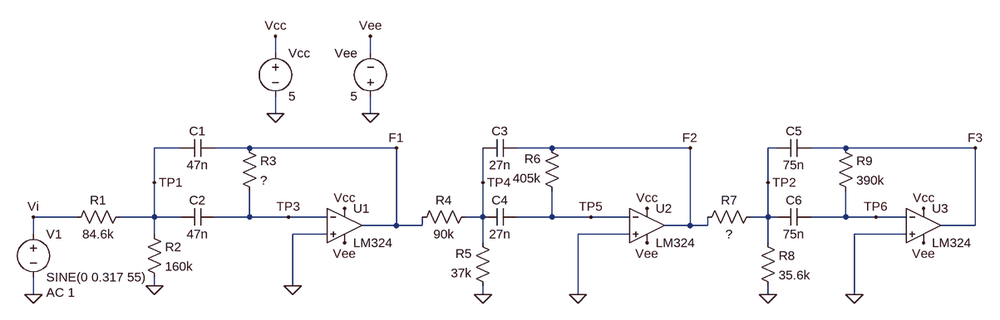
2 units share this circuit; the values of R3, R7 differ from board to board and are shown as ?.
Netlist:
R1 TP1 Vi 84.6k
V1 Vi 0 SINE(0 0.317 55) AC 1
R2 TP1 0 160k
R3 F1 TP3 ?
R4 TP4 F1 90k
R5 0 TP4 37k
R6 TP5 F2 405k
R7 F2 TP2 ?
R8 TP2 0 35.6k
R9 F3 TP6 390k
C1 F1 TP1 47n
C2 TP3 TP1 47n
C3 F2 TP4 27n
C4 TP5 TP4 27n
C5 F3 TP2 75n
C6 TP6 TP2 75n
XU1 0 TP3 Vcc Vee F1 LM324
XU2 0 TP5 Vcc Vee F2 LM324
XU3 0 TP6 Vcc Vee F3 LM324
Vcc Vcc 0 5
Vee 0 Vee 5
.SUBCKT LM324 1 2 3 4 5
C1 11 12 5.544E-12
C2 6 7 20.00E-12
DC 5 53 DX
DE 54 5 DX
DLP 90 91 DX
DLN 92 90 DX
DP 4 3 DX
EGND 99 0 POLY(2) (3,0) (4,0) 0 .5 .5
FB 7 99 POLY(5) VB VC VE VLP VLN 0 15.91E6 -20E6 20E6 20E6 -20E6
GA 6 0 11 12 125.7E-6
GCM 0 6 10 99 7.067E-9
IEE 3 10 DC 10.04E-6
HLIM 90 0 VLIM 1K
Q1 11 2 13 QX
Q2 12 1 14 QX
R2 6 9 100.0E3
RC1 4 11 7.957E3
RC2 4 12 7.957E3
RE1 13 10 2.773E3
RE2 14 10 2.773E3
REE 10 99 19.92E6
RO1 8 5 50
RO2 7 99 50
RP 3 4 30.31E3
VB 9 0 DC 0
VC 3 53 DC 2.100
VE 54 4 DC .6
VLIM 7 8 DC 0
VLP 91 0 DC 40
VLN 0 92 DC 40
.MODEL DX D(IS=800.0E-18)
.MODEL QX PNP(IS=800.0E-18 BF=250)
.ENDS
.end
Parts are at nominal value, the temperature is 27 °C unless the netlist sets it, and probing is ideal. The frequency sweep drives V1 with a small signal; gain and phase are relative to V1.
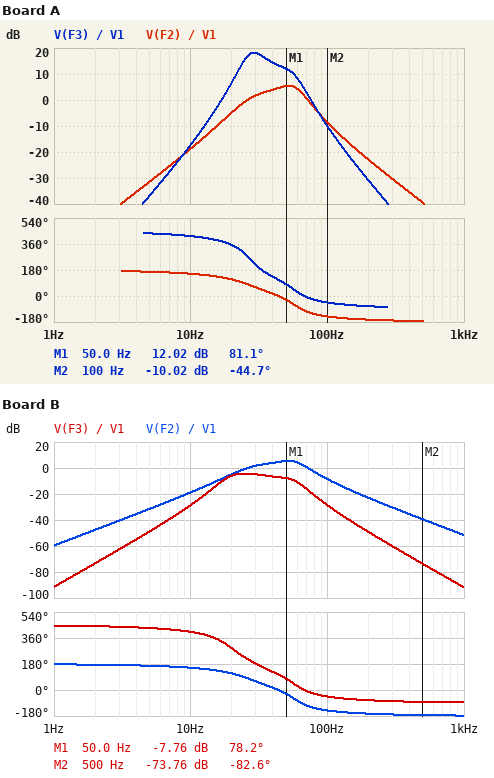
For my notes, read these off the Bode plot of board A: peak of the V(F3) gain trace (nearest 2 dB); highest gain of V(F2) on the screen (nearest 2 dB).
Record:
18 dB
6 dB
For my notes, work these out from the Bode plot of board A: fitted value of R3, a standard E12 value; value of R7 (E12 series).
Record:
270 kΩ
27 kΩ
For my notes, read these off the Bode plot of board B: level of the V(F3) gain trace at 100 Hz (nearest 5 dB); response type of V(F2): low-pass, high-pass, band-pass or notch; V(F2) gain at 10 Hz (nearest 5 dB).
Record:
-30 dB
band-pass
-20 dB
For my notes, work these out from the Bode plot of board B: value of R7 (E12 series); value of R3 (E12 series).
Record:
220 kΩ
270 kΩ
